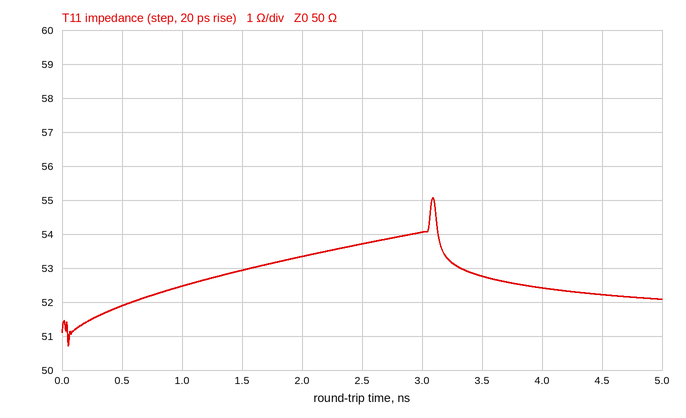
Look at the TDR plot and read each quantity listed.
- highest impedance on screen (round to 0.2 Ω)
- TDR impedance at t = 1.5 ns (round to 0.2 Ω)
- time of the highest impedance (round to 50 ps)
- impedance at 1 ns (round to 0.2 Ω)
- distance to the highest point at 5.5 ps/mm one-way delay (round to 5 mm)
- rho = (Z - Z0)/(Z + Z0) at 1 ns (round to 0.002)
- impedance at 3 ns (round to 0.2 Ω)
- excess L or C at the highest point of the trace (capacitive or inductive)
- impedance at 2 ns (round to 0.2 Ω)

55.0 Ω
53.0 Ω
3.10 ns
52.4 Ω
280 mm
+0.024
54.0 Ω
inductive
53.4 Ω
